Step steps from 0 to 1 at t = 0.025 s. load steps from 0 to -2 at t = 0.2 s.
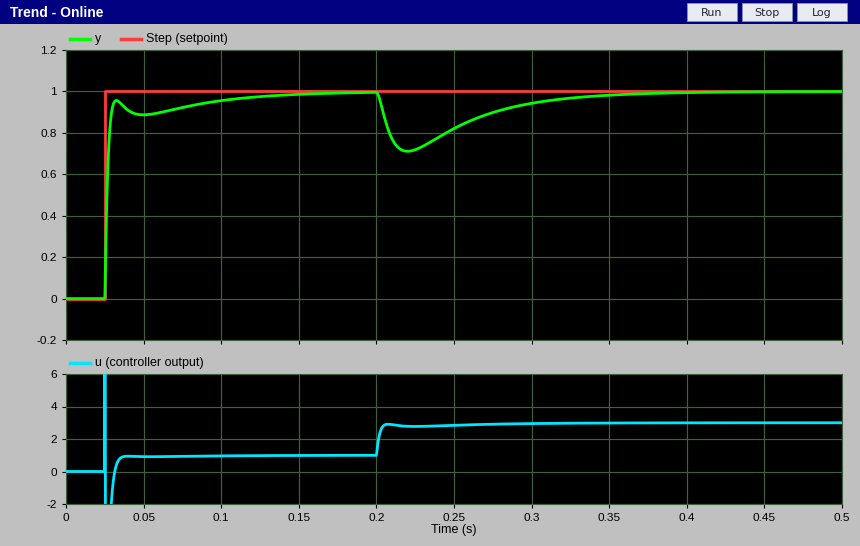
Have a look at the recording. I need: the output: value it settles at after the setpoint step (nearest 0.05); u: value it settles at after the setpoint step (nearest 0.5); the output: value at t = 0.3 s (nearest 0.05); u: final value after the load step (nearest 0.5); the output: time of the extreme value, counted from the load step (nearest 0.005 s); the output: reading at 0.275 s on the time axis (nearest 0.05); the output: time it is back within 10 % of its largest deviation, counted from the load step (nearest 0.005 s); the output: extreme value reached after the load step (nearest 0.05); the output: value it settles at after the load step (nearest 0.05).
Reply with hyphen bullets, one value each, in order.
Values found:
- 1.00
- 1.0
- 0.95
- 3.0
- 0.020 s
- 0.90
- 0.130 s
- 0.70
- 1.00
